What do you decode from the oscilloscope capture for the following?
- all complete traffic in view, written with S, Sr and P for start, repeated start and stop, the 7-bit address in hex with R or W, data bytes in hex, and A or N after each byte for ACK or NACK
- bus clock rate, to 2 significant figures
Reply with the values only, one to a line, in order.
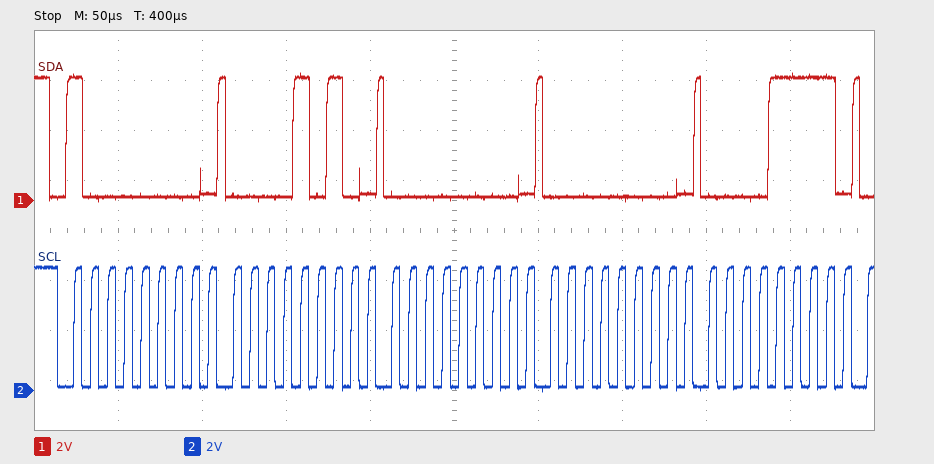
S 40W A 0A A 00 A 00 A 0F A
100 kHz
